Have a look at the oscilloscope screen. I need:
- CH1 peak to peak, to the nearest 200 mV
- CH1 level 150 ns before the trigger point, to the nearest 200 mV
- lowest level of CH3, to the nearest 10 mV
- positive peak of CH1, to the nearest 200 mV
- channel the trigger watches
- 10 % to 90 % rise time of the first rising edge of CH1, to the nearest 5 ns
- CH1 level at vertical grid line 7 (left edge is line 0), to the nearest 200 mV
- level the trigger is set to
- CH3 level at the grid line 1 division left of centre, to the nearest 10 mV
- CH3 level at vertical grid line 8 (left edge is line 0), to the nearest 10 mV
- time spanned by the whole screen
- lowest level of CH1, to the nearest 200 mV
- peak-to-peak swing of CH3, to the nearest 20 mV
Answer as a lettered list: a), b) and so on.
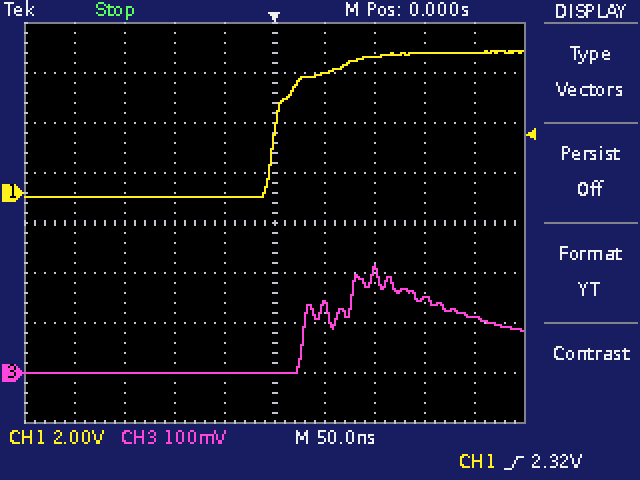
a) 5.8 V
b) -200 mV
c) 0 mV
d) 5.6 V
e) CH1
f) 75 ns
g) 5.4 V
h) 2.32 V
i) 0 mV
j) 150 mV
k) 500 ns
l) -200 mV
m) 220 mV
